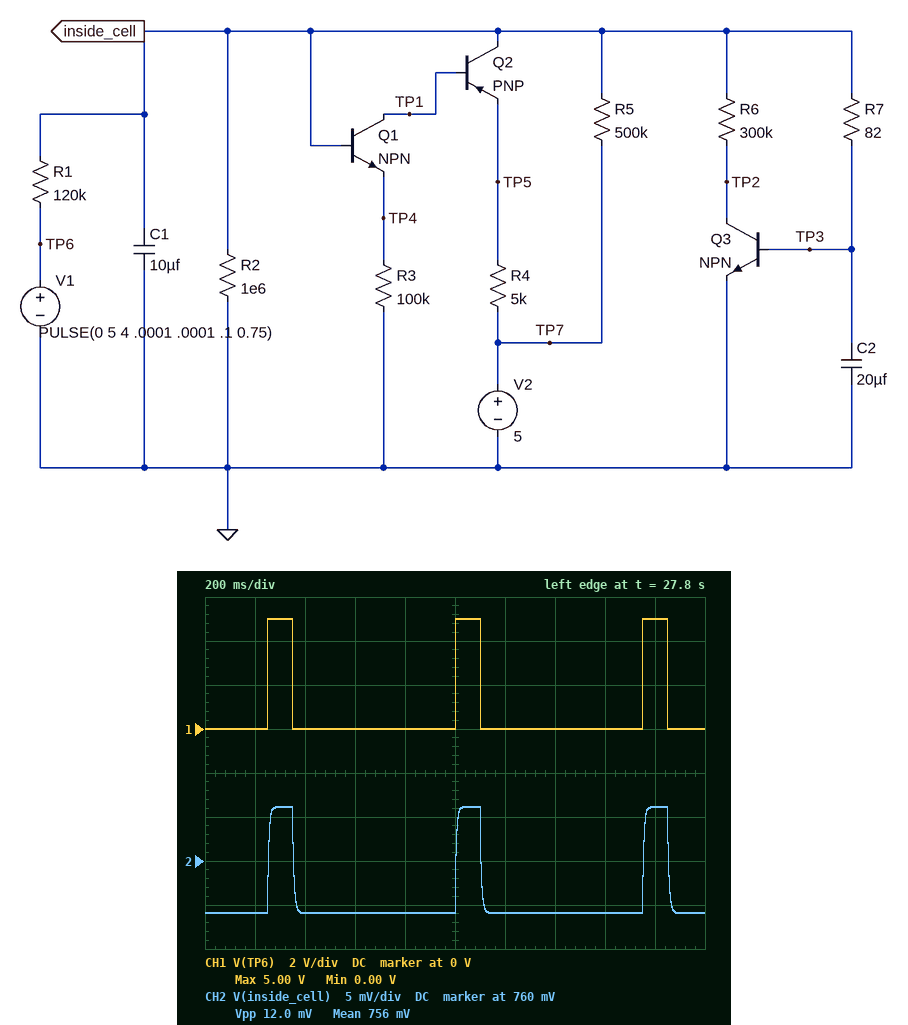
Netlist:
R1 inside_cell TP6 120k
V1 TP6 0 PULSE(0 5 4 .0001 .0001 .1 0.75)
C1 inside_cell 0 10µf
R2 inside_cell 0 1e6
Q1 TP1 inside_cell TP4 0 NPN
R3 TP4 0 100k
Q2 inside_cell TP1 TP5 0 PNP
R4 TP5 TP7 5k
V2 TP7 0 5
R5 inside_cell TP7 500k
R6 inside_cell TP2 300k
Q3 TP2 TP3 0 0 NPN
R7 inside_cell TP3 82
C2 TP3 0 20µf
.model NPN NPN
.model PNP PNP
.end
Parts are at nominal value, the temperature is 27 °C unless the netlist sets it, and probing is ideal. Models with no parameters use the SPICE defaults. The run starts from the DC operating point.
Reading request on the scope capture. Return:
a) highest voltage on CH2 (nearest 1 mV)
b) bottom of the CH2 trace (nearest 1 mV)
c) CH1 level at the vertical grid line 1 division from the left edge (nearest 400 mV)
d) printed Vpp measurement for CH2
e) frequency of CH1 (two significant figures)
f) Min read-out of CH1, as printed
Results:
766 mV
754 mV
0 V
12.0 mV
1.3 Hz
0.00 V
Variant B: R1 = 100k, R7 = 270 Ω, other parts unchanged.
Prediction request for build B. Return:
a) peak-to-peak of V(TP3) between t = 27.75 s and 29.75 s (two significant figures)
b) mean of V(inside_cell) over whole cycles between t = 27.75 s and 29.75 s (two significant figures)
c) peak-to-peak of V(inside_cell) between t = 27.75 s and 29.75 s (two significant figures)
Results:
9.0 mV
800 mV
29 mV
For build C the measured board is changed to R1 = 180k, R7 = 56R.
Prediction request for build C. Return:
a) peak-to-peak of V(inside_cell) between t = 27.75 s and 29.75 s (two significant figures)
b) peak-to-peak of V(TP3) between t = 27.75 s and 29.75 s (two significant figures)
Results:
7.3 mV
5.4 mV
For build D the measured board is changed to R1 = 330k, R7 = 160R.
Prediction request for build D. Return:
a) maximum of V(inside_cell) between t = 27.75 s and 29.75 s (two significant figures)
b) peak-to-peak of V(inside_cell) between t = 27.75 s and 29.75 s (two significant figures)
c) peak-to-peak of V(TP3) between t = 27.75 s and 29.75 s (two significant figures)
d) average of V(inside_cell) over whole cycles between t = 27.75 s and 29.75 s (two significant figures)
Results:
780 mV
6.3 mV
3.0 mV
770 mV
